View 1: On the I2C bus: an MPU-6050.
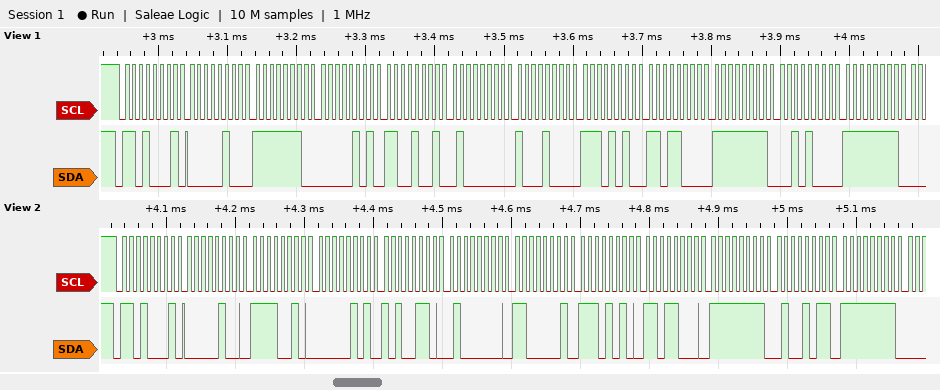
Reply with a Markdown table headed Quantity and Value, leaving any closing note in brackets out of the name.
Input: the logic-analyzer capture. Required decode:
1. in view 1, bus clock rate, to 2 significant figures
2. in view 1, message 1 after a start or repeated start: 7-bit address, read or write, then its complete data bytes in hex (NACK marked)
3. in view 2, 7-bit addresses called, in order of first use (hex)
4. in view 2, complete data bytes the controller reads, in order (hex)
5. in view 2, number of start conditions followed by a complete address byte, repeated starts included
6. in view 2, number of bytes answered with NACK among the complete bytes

| Quantity | Value |
|---|---|
| in view 1, bus clock rate, to 2 significant figures | 100 kHz |
| in view 1, message 1 after a start or repeated start: 7-bit address, read or write, then its complete data bytes in hex | 0x68 read: 04 FE 05 C9 40 88 EA D8 FF 28 FF |
| in view 2, 7-bit addresses called, in order of first use | 0x68 |
| in view 2, complete data bytes the controller reads, in order | 04 F2 05 A6 40 C1 EA D8 FF 4B FF |
| in view 2, number of start conditions followed by a complete address byte, repeated starts included | 1 |
| in view 2, number of bytes answered with NACK among the complete bytes | 0 |
